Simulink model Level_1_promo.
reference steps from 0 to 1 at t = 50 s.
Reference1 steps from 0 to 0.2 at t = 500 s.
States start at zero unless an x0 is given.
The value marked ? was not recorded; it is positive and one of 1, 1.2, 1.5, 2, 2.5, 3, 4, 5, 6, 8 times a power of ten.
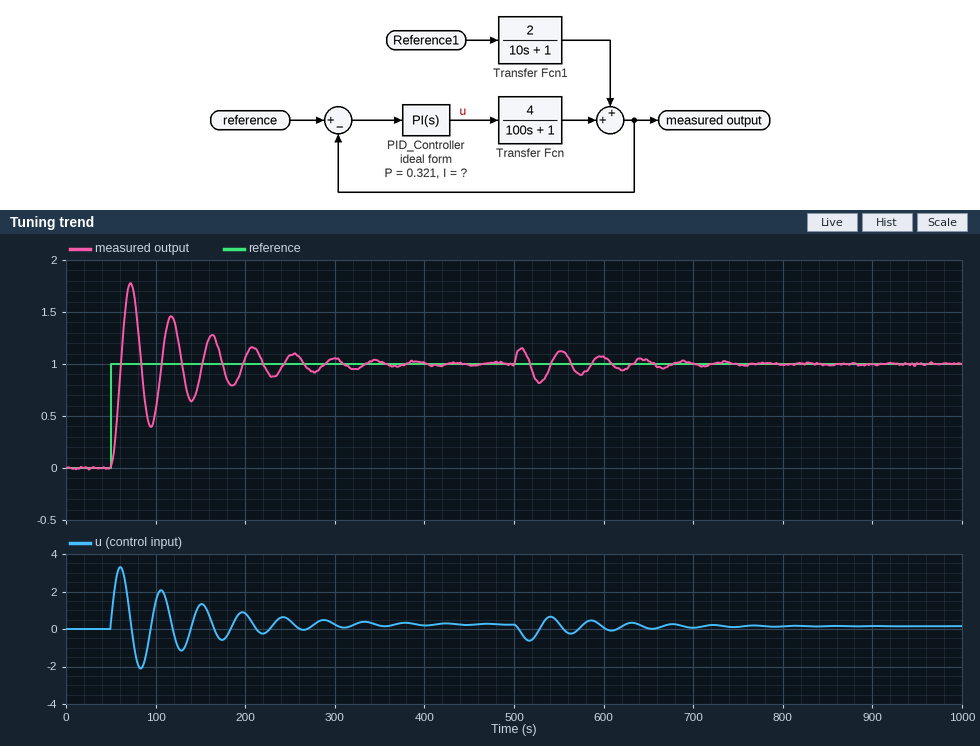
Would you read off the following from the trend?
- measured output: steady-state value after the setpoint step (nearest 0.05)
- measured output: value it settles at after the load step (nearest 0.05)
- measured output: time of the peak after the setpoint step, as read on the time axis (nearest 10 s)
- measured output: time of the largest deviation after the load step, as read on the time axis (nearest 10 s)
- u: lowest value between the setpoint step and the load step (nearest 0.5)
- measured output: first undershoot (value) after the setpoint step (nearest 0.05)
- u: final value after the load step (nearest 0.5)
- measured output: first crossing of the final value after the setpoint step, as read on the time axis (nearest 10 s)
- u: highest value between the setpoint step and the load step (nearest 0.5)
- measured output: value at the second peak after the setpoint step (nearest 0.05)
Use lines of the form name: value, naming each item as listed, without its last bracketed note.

measured output: steady-state value after the setpoint step: 1.00
measured output: value it settles at after the load step: 1.00
measured output: time of the peak after the setpoint step, as read on the time axis: 70 s
measured output: time of the largest deviation after the load step, as read on the time axis: 530 s
u: lowest value between the setpoint step and the load step: -2.0
measured output: first undershoot (value) after the setpoint step: 0.40
u: final value after the load step: 0.0
measured output: first crossing of the final value after the setpoint step, as read on the time axis: 60 s
u: highest value between the setpoint step and the load step: 3.5
measured output: value at the second peak after the setpoint step: 1.45
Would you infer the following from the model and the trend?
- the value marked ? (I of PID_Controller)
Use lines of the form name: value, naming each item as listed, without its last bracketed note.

the value marked ?: 1.5
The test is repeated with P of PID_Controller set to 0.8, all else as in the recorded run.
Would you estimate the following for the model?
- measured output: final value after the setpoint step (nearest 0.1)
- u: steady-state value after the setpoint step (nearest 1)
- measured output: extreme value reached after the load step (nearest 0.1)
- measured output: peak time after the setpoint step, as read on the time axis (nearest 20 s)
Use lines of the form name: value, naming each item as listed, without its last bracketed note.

measured output: final value after the setpoint step: 1.0
u: steady-state value after the setpoint step: 0
measured output: extreme value reached after the load step: 0.9
measured output: peak time after the setpoint step, as read on the time axis: 60 s
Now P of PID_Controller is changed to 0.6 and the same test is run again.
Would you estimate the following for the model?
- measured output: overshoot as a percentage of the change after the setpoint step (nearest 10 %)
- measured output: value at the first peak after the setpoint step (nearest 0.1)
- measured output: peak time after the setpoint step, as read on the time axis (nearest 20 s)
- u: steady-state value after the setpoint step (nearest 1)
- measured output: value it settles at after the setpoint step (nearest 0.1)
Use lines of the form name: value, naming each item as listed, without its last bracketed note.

measured output: overshoot as a percentage of the change after the setpoint step: 80 %
measured output: value at the first peak after the setpoint step: 1.8
measured output: peak time after the setpoint step, as read on the time axis: 60 s
u: steady-state value after the setpoint step: 0
measured output: value it settles at after the setpoint step: 1.0
